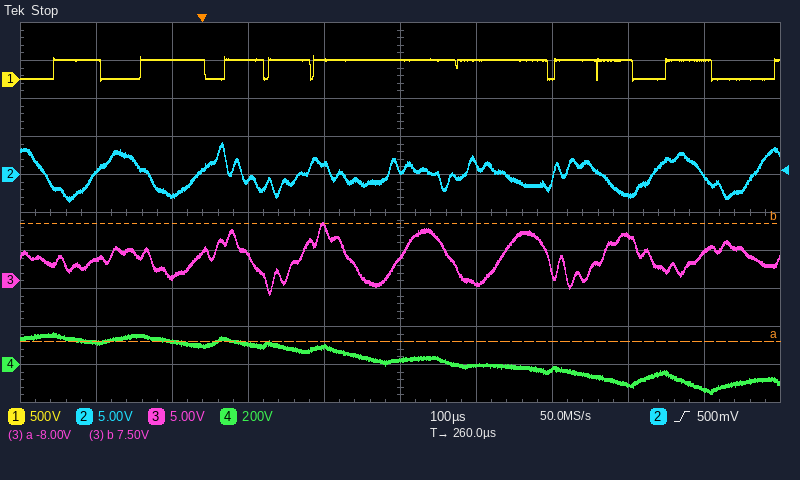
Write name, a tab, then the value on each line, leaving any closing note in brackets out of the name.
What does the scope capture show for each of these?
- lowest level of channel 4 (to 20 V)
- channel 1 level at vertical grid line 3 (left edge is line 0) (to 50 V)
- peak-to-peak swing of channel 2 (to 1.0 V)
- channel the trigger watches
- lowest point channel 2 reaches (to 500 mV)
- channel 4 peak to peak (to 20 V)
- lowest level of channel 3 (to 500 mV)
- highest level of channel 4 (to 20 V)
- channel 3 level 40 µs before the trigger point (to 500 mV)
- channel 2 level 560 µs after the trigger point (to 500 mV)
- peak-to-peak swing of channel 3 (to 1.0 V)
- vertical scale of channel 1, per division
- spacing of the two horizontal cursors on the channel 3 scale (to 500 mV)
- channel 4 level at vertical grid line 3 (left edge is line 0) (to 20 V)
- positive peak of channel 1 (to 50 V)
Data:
lowest level of channel 4	-160 V
channel 1 level at vertical grid line 3 (left edge is line 0)	250 V
peak-to-peak swing of channel 2	8.0 V
channel the trigger watches	channel 2
lowest point channel 2 reaches	-3.5 V
channel 4 peak to peak	320 V
lowest level of channel 3	-2.0 V
highest level of channel 4	160 V
channel 3 level 40 µs before the trigger point	500 mV
channel 2 level 560 µs after the trigger point	-3.0 V
peak-to-peak swing of channel 3	10.0 V
vertical scale of channel 1, per division	500 V
spacing of the two horizontal cursors on the channel 3 scale	15.5 V
channel 4 level at vertical grid line 3 (left edge is line 0)	100 V
positive peak of channel 1	300 V
